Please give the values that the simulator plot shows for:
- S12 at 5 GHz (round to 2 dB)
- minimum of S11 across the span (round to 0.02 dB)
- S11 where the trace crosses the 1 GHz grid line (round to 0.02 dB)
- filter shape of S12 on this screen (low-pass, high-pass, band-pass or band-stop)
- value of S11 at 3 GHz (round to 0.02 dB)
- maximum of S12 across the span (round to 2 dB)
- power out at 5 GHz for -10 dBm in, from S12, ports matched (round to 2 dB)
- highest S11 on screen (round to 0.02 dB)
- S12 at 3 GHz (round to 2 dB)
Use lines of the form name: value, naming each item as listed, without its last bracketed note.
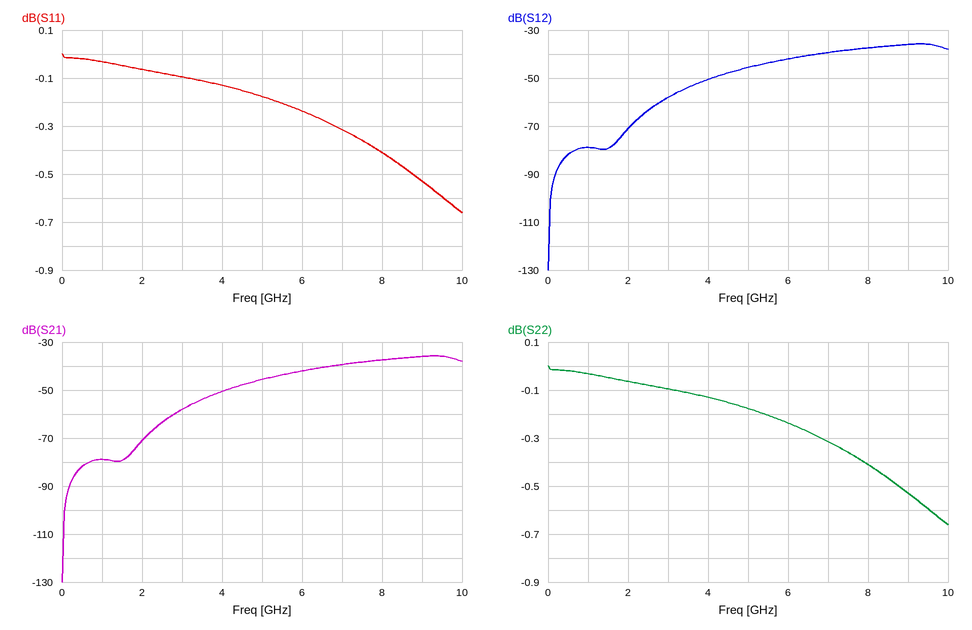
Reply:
S12 at 5 GHz: -46 dB
minimum of S11 across the span: -0.66 dB
S11 where the trace crosses the 1 GHz grid line: -0.04 dB
filter shape of S12 on this screen: high-pass
value of S11 at 3 GHz: -0.10 dB
maximum of S12 across the span: -36 dB
power out at 5 GHz for -10 dBm in, from S12, ports matched: -56 dBm
highest S11 on screen: 0.00 dB
S12 at 3 GHz: -58 dB
